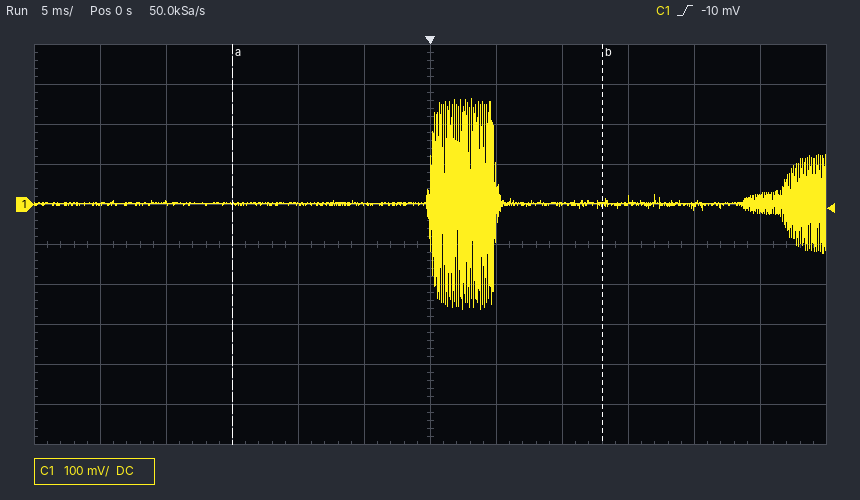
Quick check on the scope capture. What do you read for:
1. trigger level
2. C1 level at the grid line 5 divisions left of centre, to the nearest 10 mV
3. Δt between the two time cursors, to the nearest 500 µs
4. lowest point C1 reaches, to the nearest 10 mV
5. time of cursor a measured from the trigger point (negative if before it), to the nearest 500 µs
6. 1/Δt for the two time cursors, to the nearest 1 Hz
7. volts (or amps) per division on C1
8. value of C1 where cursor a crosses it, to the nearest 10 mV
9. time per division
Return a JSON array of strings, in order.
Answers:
["-10 mV", "0 mV", "28.0 ms", "-260 mV", "-15.0 ms", "36 Hz", "100 mV", "0 mV", "5 ms"]
